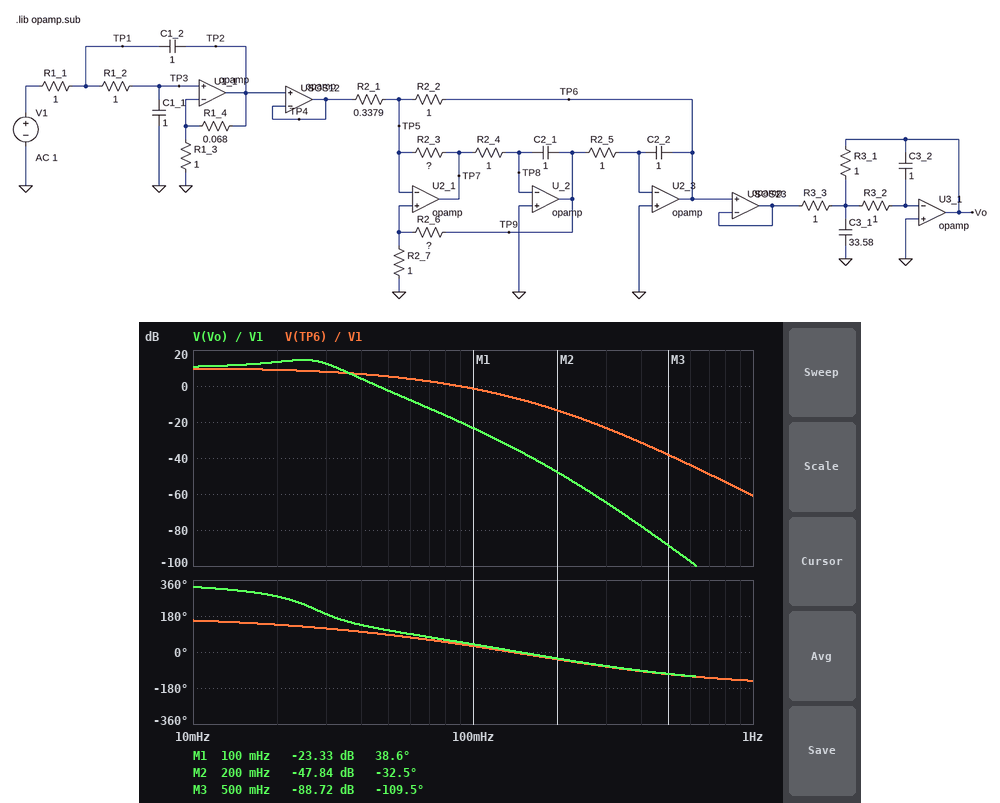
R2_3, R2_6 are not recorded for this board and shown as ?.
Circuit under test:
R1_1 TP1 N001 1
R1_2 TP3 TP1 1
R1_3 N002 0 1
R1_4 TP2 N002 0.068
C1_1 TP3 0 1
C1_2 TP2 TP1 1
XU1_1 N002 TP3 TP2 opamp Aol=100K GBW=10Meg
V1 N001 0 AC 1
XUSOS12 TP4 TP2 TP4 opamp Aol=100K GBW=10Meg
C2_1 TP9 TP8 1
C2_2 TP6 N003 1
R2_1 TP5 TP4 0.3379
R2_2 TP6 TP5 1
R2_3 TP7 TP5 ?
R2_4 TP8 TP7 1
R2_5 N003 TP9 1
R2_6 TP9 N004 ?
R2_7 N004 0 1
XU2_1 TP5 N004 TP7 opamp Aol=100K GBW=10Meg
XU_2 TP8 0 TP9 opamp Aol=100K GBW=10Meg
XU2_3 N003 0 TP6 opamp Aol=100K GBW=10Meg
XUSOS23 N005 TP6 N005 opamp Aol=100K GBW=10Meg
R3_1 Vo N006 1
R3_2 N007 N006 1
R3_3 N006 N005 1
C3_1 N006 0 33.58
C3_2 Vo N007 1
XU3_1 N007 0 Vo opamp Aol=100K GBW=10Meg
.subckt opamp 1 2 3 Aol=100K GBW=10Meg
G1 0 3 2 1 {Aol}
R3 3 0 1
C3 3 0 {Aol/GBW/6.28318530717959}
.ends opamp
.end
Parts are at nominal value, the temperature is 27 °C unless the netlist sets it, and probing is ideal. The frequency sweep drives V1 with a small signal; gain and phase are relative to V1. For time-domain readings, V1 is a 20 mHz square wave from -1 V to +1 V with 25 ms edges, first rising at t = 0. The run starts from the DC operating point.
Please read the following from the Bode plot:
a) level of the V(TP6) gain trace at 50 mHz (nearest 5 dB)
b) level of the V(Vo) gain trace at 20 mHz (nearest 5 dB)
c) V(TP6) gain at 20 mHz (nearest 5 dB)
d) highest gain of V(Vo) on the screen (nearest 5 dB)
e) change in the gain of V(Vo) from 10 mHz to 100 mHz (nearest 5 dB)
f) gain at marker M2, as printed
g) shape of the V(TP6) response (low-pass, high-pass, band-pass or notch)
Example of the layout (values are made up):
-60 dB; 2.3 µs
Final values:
5 dB; 15 dB; 10 dB; 15 dB; -35 dB; -47.84 dB; low-pass
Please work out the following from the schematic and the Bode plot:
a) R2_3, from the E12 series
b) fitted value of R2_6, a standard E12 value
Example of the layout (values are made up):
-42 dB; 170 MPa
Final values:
0.47 Ω; 0.39 Ω
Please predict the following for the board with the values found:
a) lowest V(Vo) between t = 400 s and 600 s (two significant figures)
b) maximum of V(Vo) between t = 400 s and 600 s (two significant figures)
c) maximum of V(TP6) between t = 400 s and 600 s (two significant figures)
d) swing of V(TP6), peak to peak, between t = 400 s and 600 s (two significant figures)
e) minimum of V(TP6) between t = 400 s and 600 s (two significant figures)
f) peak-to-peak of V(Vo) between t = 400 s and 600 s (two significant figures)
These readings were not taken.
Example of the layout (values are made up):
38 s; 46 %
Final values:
-5.8 V; 5.8 V; 3.1 V; 6.3 V; -3.1 V; 12 V
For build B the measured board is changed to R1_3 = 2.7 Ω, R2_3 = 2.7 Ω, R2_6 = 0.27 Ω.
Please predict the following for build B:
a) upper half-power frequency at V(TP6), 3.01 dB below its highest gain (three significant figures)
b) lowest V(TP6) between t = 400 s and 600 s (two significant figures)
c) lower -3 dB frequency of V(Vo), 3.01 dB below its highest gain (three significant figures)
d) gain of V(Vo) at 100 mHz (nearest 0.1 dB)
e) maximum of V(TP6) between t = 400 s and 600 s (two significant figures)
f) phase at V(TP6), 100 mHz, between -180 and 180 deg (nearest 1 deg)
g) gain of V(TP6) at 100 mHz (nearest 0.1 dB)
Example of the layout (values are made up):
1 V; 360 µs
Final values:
42.0 mHz; -3.0 V; 14.3 mHz; -22.3 dB; 3.0 V; 48 deg; -0.4 dB
